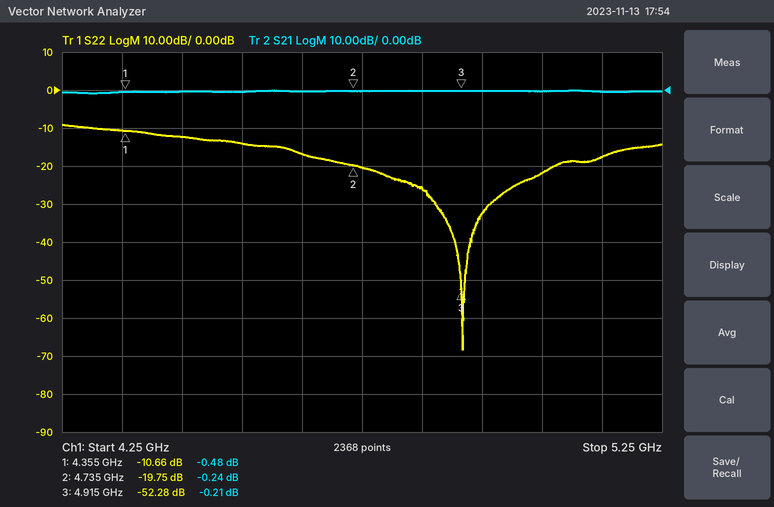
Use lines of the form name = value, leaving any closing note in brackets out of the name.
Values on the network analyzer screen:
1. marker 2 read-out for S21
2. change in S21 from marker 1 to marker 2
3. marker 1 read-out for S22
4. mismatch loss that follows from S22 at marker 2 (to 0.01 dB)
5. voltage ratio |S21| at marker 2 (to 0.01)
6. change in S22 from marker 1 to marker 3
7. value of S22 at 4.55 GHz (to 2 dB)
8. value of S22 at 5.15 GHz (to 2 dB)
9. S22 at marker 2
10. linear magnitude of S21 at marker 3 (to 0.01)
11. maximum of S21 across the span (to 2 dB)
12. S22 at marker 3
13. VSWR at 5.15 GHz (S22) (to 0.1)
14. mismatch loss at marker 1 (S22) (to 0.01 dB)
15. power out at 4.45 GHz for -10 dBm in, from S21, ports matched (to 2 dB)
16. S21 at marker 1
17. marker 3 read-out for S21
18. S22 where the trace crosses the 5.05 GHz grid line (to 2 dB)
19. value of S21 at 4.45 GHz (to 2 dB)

marker 2 read-out for S21 = -0.24 dB
change in S21 from marker 1 to marker 2 = 0.24 dB
marker 1 read-out for S22 = -10.66 dB
mismatch loss that follows from S22 at marker 2 = 0.05 dB
voltage ratio |S21| at marker 2 = 0.97
change in S22 from marker 1 to marker 3 = -41.62 dB
value of S22 at 4.55 GHz = -14 dB
value of S22 at 5.15 GHz = -18 dB
S22 at marker 2 = -19.75 dB
linear magnitude of S21 at marker 3 = 0.98
maximum of S21 across the span = 0 dB
S22 at marker 3 = -52.28 dB
VSWR at 5.15 GHz (S22) = 1.3
mismatch loss at marker 1 (S22) = 0.39 dB
power out at 4.45 GHz for -10 dBm in, from S21, ports matched = -10 dBm
S21 at marker 1 = -0.48 dB
marker 3 read-out for S21 = -0.21 dB
S22 where the trace crosses the 5.05 GHz grid line = -22 dB
value of S21 at 4.45 GHz = 0 dB
